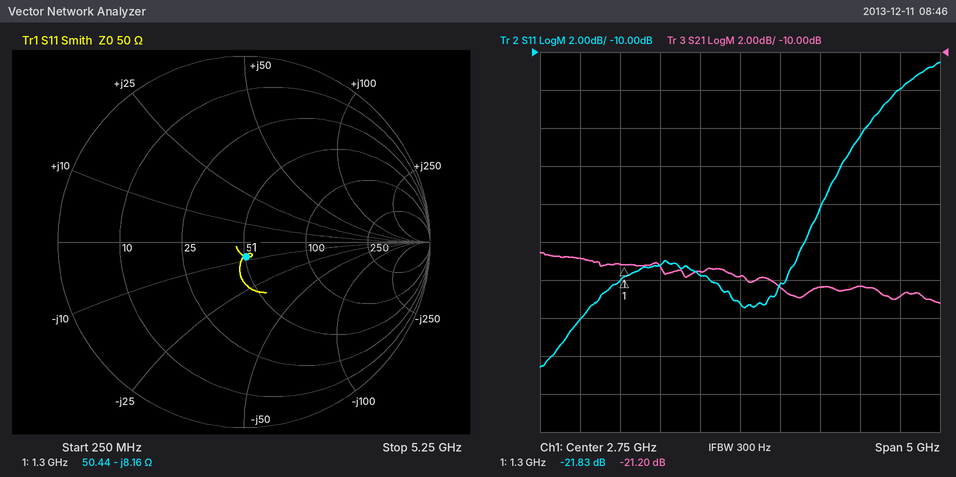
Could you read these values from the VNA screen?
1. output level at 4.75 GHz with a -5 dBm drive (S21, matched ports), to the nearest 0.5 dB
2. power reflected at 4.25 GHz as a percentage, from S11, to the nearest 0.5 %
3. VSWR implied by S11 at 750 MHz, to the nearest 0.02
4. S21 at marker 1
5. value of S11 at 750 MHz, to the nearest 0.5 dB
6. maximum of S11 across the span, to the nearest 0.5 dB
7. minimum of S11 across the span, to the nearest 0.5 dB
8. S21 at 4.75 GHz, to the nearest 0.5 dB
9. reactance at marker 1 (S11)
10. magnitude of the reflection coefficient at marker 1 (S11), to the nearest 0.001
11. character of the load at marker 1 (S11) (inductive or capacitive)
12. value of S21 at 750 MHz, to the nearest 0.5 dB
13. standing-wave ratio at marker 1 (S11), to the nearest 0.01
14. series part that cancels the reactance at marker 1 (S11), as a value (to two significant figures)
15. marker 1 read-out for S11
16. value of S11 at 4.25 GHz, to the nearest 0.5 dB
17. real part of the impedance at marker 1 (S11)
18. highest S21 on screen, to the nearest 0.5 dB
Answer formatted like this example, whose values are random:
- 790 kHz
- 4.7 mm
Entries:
- -28.0 dBm
- 3.5 %
- 1.14
- -21.20 dB
- -24.0 dB
- -10.5 dB
- -26.5 dB
- -23.0 dB
- -8.16 Ω
- 0.081
- capacitive
- -21.0 dB
- 1.18
- 1.00 nH
- -21.83 dB
- -14.5 dB
- 50.44 Ω
- -20.5 dB
